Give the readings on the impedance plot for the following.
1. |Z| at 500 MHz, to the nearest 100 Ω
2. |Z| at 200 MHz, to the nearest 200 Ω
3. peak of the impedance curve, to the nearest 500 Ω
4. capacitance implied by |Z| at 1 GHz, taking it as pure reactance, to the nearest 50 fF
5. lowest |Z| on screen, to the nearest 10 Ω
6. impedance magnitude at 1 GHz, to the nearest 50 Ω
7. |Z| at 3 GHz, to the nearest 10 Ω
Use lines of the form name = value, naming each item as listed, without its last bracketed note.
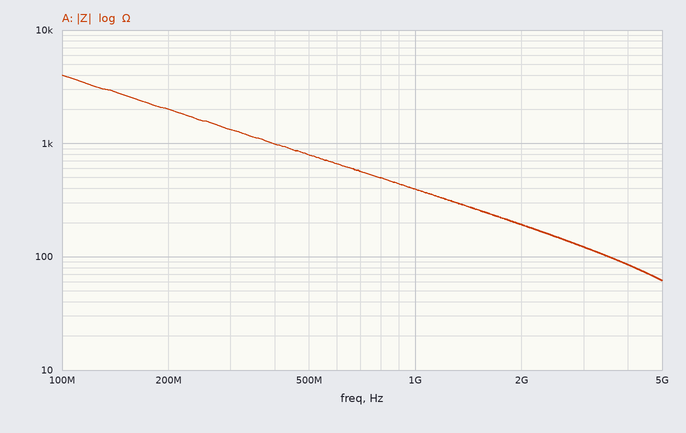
|Z| at 500 MHz, to the nearest 100 Ω = 800 Ω
|Z| at 200 MHz, to the nearest 200 Ω = 2.0 kΩ
peak of the impedance curve, to the nearest 500 Ω = 4.0 kΩ
capacitance implied by |Z| at 1 GHz, taking it as pure reactance, to the nearest 50 fF = 400 fF
lowest |Z| on screen, to the nearest 10 Ω = 60 Ω
impedance magnitude at 1 GHz, to the nearest 50 Ω = 400 Ω
|Z| at 3 GHz, to the nearest 10 Ω = 120 Ω
